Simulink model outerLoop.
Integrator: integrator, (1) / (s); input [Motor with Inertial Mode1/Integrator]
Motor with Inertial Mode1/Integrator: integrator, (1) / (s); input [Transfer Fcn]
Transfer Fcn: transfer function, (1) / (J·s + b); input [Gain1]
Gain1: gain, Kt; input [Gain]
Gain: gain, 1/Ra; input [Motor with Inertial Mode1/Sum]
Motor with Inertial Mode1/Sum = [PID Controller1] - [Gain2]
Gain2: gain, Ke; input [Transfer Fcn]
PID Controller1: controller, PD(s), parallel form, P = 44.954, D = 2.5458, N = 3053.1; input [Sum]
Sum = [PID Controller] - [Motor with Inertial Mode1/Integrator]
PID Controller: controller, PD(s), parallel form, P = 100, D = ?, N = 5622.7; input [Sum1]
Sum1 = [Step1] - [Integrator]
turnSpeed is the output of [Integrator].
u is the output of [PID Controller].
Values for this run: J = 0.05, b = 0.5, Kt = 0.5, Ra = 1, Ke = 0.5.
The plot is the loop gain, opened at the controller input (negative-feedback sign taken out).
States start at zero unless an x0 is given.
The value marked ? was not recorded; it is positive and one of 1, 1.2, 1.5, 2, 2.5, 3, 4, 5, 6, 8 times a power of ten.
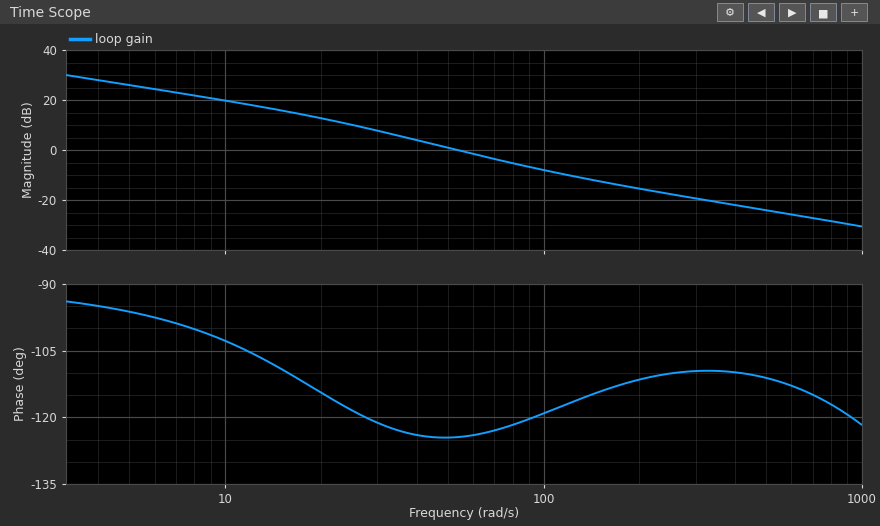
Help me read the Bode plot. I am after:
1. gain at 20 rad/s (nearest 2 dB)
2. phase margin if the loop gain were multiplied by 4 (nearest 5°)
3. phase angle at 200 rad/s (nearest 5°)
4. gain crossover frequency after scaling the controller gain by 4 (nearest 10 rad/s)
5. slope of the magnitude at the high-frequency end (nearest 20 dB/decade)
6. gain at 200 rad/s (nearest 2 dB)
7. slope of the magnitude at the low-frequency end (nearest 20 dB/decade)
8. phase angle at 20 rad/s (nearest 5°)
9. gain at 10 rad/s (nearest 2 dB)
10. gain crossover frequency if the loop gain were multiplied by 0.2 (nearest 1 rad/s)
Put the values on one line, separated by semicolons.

12 dB; 65°; -110°; 140 rad/s; -20 dB/decade; -16 dB; -20 dB/decade; -115°; 20 dB; 18 rad/s
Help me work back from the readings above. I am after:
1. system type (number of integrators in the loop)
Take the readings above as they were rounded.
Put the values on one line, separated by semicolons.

1
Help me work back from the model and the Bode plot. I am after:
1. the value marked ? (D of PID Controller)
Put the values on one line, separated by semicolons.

1.2
